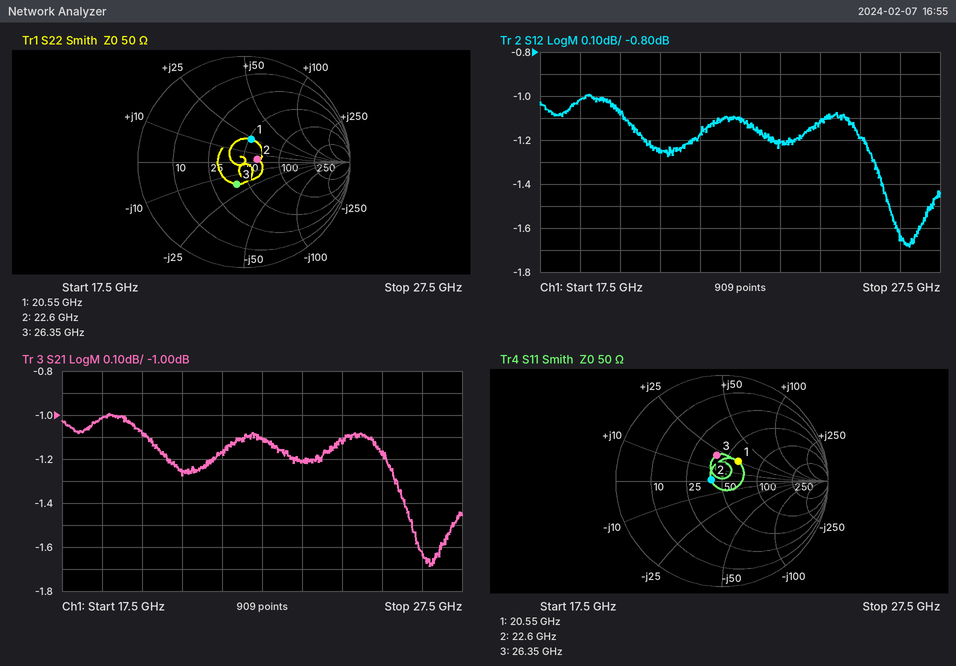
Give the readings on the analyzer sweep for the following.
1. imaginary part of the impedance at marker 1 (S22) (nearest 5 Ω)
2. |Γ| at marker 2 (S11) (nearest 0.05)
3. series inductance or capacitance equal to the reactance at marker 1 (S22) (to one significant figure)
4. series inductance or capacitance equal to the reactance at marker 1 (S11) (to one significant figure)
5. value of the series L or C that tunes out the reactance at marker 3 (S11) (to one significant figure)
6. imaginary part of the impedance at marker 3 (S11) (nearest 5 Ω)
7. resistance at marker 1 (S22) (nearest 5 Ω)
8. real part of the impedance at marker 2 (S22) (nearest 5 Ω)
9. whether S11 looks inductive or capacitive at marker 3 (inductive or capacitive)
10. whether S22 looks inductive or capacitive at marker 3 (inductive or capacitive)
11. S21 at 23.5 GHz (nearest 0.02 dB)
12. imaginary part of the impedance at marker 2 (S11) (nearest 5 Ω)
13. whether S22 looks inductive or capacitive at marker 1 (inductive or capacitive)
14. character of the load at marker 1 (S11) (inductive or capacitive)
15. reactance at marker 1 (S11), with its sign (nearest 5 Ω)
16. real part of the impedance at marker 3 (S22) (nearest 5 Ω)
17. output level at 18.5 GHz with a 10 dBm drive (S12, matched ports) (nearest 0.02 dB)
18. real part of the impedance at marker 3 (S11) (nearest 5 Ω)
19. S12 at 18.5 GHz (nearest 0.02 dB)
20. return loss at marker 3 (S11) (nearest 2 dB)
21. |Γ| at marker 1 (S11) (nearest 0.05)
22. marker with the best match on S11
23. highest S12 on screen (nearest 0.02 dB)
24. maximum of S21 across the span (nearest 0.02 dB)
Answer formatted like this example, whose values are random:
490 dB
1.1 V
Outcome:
+25 Ω
0.10
200 pH
200 pH
300 fF
+20 Ω
50 Ω
65 Ω
inductive
capacitive
-1.20 dB
0 Ω
inductive
inductive
+25 Ω
40 Ω
8.98 dBm
40 Ω
-1.02 dB
12 dB
0.25
marker 2
-1.00 dB
-1.00 dB
